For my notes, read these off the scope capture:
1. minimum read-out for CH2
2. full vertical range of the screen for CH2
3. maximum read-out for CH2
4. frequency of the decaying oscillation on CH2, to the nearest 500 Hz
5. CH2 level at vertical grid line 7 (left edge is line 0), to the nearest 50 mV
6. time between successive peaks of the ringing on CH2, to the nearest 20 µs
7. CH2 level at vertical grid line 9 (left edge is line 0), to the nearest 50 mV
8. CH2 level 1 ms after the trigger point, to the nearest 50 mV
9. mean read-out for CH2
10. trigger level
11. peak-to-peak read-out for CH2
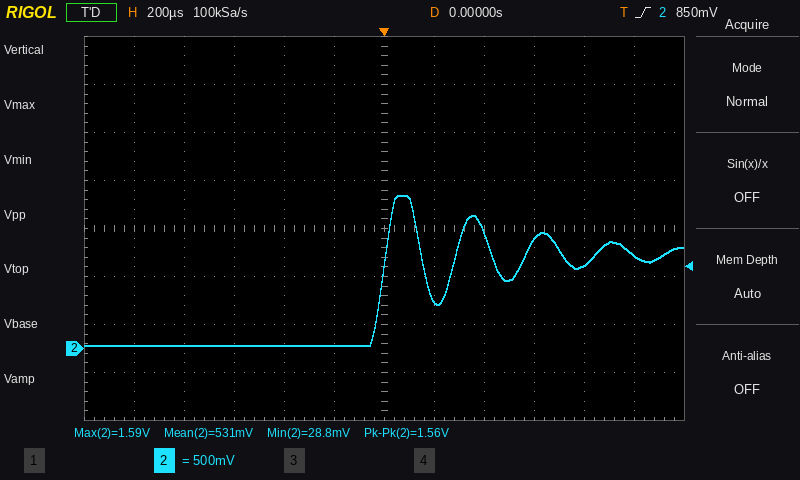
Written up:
28.8 mV
4 V
1.59 V
3.5 kHz
500 mV
280 µs
1.15 V
950 mV
531 mV
850 mV
1.56 V
